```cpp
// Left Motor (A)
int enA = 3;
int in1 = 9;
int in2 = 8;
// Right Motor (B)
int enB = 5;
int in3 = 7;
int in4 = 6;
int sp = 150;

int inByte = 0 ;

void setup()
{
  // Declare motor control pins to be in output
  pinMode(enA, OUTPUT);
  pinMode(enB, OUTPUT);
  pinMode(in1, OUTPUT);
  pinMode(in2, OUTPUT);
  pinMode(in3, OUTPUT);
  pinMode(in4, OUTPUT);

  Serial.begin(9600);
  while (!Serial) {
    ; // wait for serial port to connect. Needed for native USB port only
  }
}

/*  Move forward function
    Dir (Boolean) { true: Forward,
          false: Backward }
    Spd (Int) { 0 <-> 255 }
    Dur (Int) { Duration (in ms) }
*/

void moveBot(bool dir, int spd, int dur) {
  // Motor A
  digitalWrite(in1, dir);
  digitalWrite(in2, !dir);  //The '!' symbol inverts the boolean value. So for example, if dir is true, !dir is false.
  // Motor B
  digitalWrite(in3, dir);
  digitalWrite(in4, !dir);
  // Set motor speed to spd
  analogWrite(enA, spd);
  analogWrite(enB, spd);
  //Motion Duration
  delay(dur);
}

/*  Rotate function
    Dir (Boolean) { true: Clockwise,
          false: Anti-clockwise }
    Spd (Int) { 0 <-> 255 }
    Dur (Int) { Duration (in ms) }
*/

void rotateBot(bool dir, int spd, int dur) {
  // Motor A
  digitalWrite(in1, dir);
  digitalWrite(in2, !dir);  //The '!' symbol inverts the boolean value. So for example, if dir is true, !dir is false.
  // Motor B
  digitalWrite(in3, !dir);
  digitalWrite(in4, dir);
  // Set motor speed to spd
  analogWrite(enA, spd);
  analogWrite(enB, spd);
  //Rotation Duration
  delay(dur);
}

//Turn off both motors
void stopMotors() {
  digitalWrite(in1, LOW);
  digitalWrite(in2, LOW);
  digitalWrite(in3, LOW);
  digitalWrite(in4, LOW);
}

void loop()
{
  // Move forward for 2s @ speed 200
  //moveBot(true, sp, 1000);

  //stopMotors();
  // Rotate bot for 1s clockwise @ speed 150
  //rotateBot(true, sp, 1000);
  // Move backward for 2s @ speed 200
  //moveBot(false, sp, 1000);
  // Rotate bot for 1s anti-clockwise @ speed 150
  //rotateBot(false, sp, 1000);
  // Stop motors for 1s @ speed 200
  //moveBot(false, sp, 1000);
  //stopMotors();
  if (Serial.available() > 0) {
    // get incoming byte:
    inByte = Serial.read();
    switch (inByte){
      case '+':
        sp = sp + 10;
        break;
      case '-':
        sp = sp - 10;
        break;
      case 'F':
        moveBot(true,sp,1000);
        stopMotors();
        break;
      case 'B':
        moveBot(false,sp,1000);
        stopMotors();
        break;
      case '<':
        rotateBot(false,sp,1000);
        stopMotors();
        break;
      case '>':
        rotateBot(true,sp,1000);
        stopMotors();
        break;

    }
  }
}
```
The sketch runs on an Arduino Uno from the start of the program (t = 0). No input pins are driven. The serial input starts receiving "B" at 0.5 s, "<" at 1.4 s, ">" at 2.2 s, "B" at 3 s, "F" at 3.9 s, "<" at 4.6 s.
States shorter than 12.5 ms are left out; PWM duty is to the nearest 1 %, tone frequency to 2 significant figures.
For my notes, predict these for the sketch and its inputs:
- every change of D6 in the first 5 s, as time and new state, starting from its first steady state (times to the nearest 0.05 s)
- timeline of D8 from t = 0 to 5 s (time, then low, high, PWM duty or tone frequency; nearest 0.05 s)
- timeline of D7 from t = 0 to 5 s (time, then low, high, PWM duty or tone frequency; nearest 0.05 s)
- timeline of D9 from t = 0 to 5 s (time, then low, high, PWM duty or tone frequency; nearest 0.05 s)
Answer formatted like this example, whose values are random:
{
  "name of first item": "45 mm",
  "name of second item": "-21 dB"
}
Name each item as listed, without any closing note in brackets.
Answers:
{
  "every change of D6 in the first 5 s, as time and new state, starting from its first steady state": "0 s low; 0.5 s high; 1.5 s low; 2.5 s high; 4.5 s low",
  "timeline of D8 from t = 0 to 5 s": "0 s low; 0.5 s high; 2.5 s low; 3.5 s high; 4.5 s low",
  "timeline of D7 from t = 0 to 5 s": "0 s low; 1.5 s high; 2.5 s low; 4.5 s high",
  "timeline of D9 from t = 0 to 5 s": "0 s low; 2.5 s high; 3.5 s low; 4.5 s high"
}
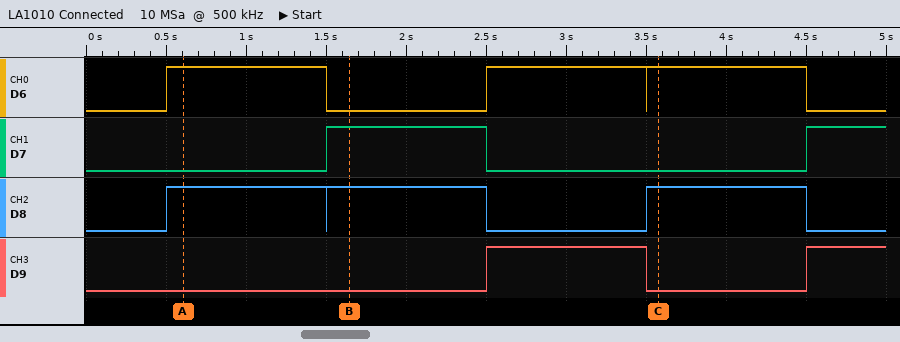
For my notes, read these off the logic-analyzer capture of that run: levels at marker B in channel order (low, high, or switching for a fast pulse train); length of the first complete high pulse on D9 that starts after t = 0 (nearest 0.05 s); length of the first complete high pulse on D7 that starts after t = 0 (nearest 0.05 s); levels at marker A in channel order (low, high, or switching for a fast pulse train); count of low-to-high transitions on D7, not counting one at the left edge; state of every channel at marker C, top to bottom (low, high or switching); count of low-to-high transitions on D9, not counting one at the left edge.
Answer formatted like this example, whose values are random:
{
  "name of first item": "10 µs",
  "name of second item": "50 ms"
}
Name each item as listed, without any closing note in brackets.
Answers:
{
  "levels at marker B in channel order": "D6 low, D7 high, D8 high, D9 low",
  "length of the first complete high pulse on D9 that starts after t = 0": "1.00 s",
  "length of the first complete high pulse on D7 that starts after t = 0": "1.00 s",
  "levels at marker A in channel order": "D6 high, D7 low, D8 high, D9 low",
  "count of low-to-high transitions on D7, not counting one at the left edge": "2",
  "state of every channel at marker C, top to bottom": "D6 high, D7 low, D8 high, D9 low",
  "count of low-to-high transitions on D9, not counting one at the left edge": "2"
}
